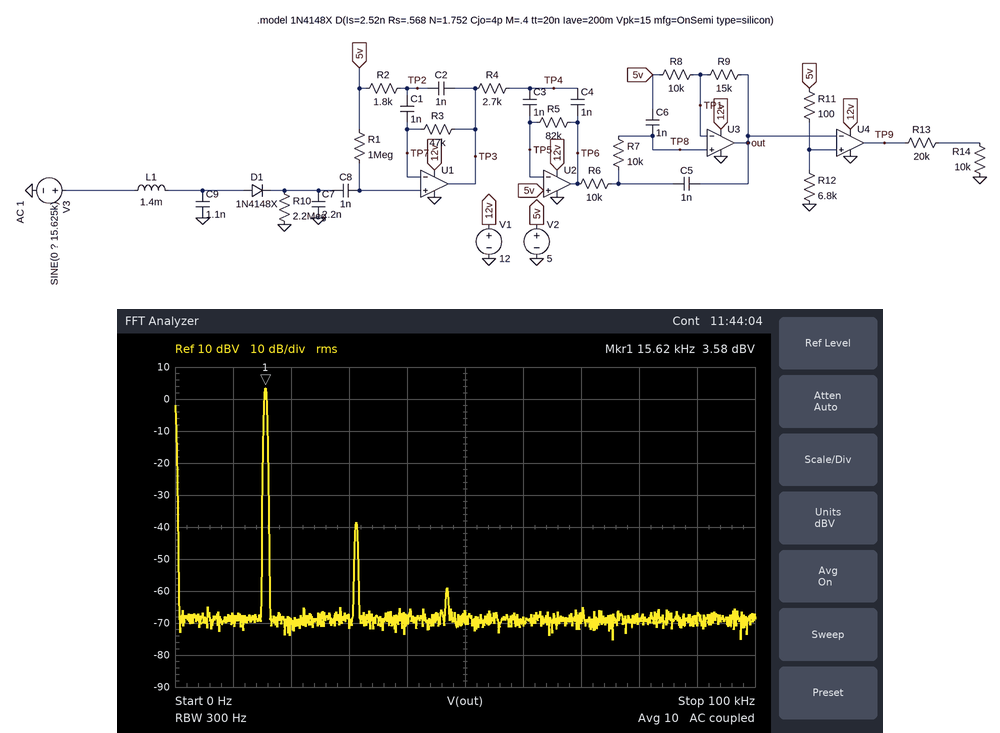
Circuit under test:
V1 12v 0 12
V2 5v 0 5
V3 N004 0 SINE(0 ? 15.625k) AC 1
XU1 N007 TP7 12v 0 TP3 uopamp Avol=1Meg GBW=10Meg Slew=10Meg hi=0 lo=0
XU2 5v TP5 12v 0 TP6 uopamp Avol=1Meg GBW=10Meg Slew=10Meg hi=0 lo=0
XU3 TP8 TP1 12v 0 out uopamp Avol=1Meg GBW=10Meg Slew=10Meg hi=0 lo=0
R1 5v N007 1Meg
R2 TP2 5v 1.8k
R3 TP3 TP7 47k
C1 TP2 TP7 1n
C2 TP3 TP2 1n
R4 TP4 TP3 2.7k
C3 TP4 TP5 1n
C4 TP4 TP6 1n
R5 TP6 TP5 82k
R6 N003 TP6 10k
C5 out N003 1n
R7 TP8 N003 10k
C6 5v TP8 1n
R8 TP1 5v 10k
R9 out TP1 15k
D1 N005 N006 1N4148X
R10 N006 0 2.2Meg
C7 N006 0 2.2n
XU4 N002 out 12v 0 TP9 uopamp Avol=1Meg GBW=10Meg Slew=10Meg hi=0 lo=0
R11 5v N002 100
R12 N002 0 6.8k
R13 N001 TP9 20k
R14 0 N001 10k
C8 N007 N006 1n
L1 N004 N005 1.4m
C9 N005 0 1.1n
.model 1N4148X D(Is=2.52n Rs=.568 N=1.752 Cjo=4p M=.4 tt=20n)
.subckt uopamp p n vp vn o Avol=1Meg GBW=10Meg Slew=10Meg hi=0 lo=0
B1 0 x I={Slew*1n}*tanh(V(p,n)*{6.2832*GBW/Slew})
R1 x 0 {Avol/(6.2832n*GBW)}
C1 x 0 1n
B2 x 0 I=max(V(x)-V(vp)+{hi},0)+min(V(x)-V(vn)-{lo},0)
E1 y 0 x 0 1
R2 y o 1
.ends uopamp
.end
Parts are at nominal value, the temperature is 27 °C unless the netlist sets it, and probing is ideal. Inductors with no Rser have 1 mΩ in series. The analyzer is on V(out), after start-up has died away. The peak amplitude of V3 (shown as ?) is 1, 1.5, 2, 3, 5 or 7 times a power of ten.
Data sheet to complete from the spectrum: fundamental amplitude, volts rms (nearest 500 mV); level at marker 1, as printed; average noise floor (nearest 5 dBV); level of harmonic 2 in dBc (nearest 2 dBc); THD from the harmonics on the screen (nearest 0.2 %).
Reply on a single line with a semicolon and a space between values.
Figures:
1.5 V; 3.58 dBV; -70 dBV; -42 dBc; 0.8 %
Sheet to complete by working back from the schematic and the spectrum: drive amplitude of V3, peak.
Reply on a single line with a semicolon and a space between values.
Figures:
1.5 V
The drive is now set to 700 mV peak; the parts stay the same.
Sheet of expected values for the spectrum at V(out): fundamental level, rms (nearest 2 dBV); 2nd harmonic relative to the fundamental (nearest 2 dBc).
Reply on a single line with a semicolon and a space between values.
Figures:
-4 dBV; -44 dBc
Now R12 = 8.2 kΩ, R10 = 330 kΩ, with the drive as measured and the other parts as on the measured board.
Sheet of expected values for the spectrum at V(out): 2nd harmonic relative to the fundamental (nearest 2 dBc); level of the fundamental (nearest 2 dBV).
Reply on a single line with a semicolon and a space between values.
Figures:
-18 dBc; 14 dBV
